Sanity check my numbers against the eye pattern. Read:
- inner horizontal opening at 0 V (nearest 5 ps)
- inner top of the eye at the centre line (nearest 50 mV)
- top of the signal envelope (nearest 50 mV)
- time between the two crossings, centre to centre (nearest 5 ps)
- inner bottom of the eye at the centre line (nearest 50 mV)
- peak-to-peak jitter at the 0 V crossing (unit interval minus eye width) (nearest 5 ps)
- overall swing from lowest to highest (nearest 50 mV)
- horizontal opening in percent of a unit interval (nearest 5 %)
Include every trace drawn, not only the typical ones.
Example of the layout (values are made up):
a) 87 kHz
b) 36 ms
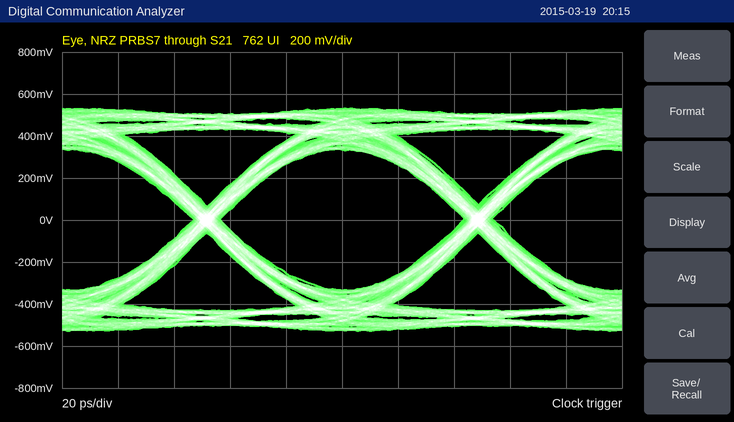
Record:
a) 85 ps
b) 350 mV
c) 550 mV
d) 95 ps
e) -350 mV
f) 10 ps
g) 1.05 V
h) 90 %
